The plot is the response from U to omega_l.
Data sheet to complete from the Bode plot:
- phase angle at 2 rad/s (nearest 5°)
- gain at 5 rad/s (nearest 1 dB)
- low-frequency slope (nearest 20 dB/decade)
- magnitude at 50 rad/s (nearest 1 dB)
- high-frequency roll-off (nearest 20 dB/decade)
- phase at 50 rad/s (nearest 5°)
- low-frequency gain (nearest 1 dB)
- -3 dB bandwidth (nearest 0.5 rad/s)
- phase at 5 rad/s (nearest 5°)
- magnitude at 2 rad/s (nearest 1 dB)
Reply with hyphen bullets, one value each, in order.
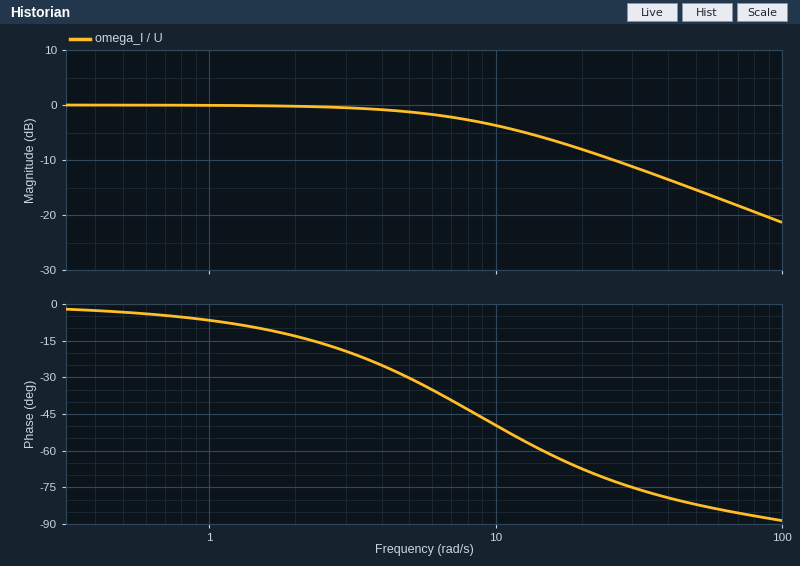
- -15°
- -1 dB
- 0 dB/decade
- -15 dB
- -20 dB/decade
- -80°
- 0 dB
- 8.5 rad/s
- -30°
- 0 dB
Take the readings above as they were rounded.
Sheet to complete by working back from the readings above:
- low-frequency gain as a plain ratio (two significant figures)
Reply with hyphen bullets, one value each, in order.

- 1.0
